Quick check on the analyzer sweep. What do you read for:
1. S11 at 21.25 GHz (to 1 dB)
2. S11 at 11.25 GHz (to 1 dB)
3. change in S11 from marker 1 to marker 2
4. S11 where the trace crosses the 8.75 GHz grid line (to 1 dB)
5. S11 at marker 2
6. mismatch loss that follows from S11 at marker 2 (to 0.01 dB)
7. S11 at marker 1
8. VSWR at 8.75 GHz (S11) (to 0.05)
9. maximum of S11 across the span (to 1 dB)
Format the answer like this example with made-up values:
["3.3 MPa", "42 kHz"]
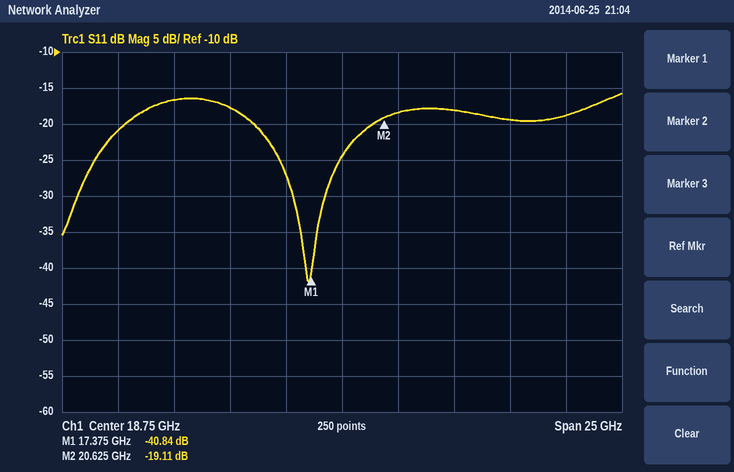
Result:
["-18 dB", "-17 dB", "21.73 dB", "-21 dB", "-19.11 dB", "0.05 dB", "-40.84 dB", "1.20", "-16 dB"]
